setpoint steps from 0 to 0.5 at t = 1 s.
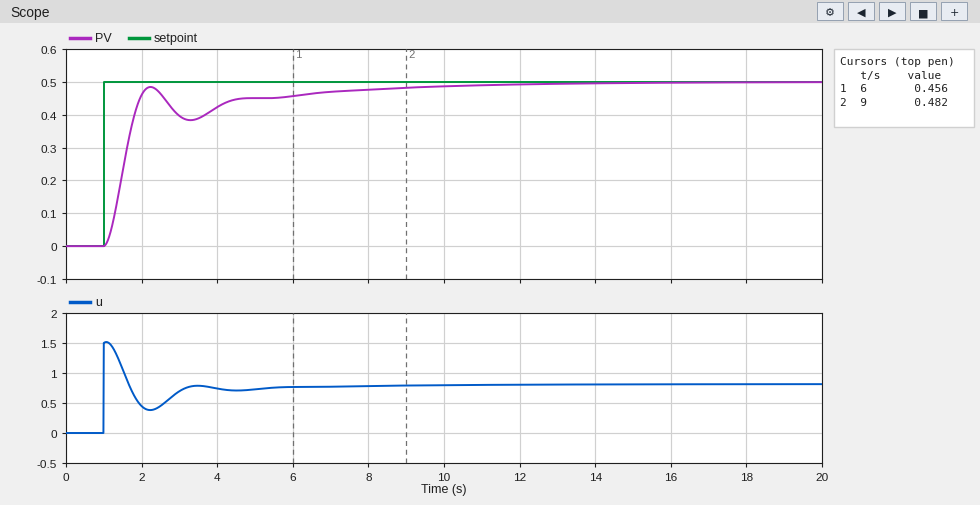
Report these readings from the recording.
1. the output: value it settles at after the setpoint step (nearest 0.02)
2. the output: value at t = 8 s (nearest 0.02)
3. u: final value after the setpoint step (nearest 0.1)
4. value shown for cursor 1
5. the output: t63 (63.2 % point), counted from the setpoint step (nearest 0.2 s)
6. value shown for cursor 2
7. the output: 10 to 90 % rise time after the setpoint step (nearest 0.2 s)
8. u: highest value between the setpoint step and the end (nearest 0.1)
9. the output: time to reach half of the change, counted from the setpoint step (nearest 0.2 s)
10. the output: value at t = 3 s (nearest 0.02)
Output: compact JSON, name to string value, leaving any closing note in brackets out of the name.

{"the output: value it settles at after the setpoint step": "0.50", "the output: value at t = 8 s": "0.48", "u: final value after the setpoint step": "0.8", "value shown for cursor 1": "0.456", "the output: t63 (63.2 % point), counted from the setpoint step": "0.6 s", "value shown for cursor 2": "0.482", "the output: 10 to 90 % rise time after the setpoint step": "0.8 s", "u: highest value between the setpoint step and the end": "1.5", "the output: time to reach half of the change, counted from the setpoint step": "0.6 s", "the output: value at t = 3 s": "0.40"}
